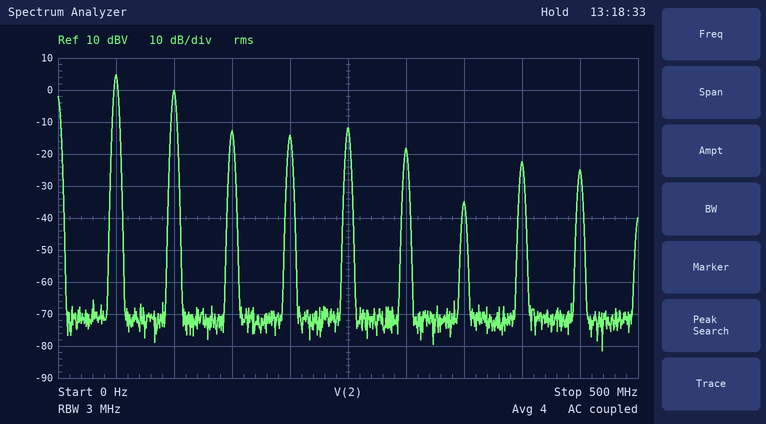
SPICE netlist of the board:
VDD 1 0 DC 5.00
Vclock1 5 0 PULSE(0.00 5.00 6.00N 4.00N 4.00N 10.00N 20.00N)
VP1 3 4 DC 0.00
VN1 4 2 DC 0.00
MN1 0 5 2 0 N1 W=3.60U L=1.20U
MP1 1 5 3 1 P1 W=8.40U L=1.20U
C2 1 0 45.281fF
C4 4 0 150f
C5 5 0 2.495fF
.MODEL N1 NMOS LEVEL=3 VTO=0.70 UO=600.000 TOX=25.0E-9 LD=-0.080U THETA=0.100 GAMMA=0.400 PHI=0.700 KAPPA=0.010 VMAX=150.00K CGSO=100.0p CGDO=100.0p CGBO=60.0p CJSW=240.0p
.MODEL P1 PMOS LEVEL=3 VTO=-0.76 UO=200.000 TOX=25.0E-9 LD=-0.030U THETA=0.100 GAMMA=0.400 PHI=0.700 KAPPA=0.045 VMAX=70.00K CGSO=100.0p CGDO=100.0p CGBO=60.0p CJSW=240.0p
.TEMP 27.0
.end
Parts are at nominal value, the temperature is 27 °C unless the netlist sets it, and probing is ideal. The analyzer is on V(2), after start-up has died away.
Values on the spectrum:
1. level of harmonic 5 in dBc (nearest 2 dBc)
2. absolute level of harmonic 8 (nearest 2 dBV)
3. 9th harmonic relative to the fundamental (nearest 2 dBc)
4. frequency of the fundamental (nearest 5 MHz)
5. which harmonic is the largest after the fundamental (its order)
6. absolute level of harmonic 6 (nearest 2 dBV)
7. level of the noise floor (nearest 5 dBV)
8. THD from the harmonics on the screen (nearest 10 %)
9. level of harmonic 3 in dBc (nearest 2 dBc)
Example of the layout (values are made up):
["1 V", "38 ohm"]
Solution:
["-16 dBc", "-22 dBV", "-30 dBc", "50 MHz", "2", "-18 dBV", "-70 dBV", "60 %", "-18 dBc"]
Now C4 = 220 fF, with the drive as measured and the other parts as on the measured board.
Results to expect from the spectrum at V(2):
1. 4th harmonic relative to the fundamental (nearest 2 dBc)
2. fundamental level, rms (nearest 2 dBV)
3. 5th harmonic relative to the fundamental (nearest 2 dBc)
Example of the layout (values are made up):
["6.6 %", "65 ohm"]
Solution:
["-20 dBc", "4 dBV", "-18 dBc"]
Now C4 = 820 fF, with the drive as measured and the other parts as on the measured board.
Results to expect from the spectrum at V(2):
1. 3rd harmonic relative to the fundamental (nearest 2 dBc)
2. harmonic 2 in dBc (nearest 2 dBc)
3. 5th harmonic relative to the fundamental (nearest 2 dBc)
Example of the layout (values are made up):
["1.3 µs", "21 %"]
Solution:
["-22 dBc", "-8 dBc", "-40 dBc"]
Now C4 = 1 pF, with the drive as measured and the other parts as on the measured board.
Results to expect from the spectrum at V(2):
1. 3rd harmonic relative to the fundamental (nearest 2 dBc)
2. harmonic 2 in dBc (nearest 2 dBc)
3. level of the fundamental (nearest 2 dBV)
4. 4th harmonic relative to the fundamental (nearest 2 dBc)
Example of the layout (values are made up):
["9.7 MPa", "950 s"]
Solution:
["-22 dBc", "-8 dBc", "0 dBV", "-40 dBc"]
